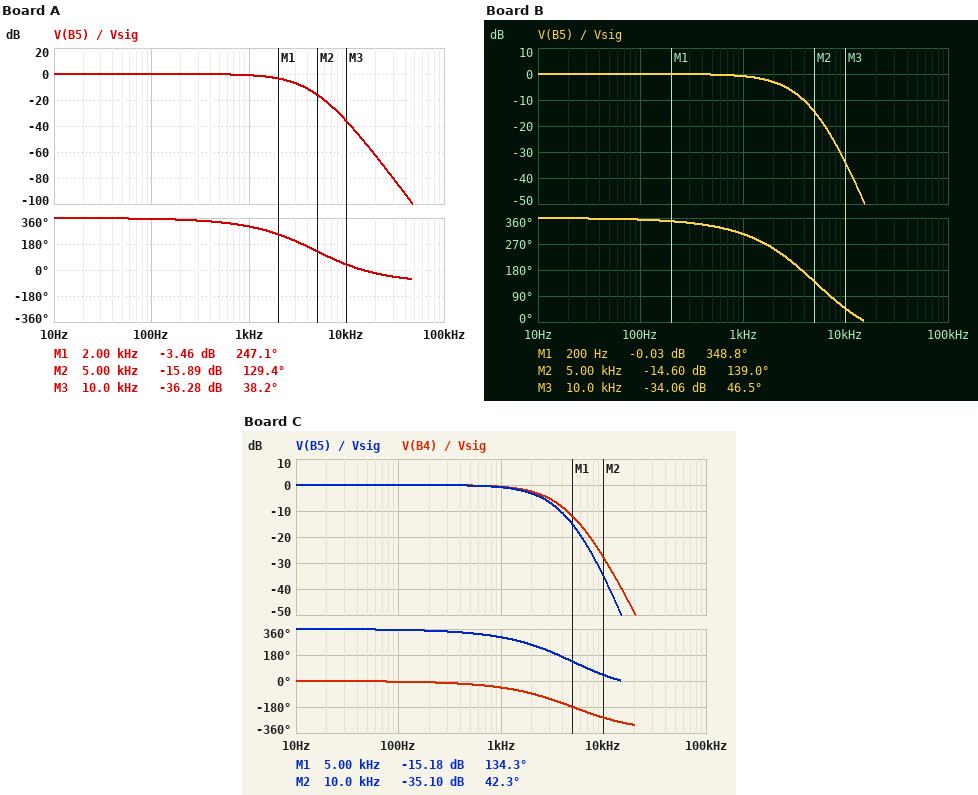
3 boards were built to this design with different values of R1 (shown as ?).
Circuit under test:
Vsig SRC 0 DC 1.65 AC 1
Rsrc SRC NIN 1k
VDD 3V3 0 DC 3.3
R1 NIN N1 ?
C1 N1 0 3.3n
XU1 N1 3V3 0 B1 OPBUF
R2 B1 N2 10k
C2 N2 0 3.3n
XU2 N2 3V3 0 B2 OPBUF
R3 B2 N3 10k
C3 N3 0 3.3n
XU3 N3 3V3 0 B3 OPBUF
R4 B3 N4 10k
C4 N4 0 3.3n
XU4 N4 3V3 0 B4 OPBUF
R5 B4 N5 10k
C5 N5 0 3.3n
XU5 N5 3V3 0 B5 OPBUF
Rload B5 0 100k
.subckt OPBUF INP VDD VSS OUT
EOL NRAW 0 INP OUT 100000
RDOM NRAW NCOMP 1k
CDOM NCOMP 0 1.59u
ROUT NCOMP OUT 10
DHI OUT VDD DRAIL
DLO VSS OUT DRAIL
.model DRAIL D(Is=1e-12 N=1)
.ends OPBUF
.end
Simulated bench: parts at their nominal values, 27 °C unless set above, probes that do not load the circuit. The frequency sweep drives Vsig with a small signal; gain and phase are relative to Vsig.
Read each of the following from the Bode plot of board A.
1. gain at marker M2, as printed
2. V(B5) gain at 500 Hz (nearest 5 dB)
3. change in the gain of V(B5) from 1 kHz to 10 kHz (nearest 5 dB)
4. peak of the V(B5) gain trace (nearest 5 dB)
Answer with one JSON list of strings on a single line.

["-15.89 dB", "0 dB", "-35 dB", "0 dB"]
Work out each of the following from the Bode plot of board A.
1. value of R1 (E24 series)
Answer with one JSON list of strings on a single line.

["9.1 kΩ"]
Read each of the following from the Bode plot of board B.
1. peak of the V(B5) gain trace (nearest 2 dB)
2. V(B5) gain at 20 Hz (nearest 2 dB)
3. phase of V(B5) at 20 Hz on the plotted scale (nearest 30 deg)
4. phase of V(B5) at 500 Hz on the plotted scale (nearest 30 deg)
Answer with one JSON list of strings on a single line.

["0 dB", "0 dB", "360 deg", "330 deg"]
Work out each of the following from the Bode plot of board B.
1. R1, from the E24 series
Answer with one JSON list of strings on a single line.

["6.2 kΩ"]
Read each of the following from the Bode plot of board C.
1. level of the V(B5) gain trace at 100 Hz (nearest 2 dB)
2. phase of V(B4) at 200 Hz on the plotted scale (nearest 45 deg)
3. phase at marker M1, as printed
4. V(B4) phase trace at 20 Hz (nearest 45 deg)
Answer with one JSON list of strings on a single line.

["0 dB", "0 deg", "134.3 deg", "0 deg"]
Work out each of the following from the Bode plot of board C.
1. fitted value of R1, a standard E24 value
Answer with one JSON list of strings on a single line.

["7.5 kΩ"]
